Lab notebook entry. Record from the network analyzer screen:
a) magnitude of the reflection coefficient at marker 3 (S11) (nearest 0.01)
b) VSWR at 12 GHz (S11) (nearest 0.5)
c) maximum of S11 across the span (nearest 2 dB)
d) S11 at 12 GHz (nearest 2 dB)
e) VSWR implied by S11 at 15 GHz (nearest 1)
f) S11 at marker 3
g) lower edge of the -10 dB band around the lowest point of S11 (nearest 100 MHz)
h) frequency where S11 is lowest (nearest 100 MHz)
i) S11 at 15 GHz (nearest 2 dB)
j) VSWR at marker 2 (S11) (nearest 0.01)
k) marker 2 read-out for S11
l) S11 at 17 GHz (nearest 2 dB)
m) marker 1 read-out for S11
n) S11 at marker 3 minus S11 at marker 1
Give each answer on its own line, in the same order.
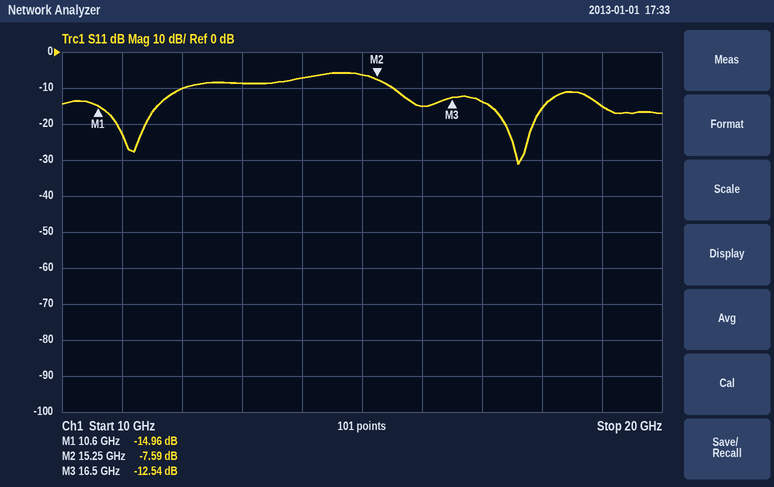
0.24
2.0
-6 dB
-10 dB
3
-12.54 dB
15.5 GHz
17.6 GHz
-6 dB
2.43
-7.59 dB
-14 dB
-14.96 dB
2.42 dB
